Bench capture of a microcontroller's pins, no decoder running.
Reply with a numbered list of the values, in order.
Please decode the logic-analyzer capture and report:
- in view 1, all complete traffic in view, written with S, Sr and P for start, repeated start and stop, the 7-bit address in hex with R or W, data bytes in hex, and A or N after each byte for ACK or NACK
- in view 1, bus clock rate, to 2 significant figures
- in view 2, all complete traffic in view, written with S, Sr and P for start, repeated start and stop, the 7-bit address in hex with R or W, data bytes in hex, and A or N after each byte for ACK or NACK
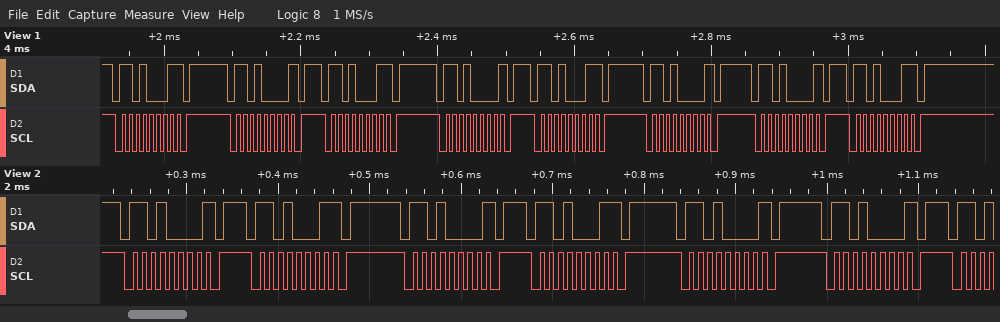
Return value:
1. S 68R N P S 68W N P S 68R N P S 68W N P S 68R N P S 68W N P S 68W N P S 68R N P
2. 100 kHz
3. S 68W N P S 68R N P S 68W N P S 68R N P S 68W N P S 68W N P
